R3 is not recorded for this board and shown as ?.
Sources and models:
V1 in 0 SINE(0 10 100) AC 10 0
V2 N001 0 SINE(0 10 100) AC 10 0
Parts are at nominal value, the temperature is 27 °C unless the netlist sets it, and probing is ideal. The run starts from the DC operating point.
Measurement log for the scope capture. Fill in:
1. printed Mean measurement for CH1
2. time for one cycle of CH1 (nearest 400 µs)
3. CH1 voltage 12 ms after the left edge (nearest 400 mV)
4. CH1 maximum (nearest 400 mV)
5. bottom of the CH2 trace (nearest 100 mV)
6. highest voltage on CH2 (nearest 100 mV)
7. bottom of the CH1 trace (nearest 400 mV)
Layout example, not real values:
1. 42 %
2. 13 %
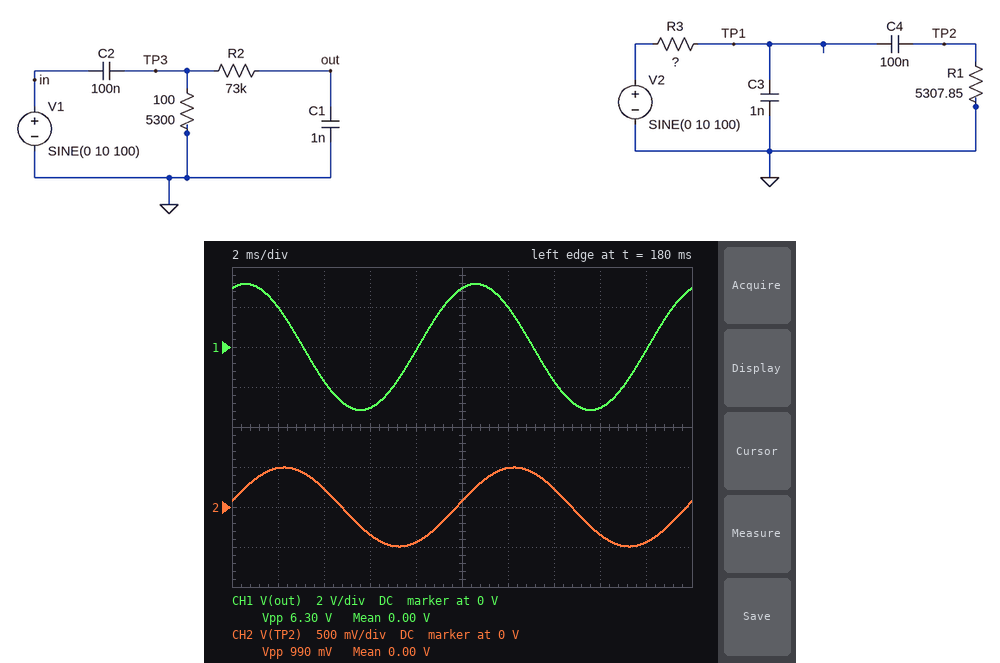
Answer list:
1. 0.00 V
2. 10.0 ms
3. 2.0 V
4. 3.2 V
5. -500 mV
6. 500 mV
7. -3.2 V
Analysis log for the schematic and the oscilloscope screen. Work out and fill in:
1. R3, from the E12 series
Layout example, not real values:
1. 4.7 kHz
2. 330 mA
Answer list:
1. 100 kΩ
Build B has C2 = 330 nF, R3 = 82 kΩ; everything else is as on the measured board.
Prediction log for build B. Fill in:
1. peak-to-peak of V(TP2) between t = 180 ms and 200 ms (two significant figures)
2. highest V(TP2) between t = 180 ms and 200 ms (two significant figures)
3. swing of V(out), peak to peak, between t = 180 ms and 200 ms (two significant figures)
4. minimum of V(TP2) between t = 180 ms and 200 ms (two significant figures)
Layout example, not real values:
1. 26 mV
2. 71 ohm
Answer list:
1. 1.2 V
2. 590 mV
3. 15 V
4. -590 mV
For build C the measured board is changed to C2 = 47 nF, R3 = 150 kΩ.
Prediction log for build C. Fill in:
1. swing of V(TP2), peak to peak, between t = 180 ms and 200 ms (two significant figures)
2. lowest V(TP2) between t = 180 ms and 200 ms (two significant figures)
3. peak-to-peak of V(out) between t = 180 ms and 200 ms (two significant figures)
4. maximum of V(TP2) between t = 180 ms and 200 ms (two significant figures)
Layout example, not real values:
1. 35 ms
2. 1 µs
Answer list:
1. 670 mV
2. -340 mV
3. 3.1 V
4. 340 mV
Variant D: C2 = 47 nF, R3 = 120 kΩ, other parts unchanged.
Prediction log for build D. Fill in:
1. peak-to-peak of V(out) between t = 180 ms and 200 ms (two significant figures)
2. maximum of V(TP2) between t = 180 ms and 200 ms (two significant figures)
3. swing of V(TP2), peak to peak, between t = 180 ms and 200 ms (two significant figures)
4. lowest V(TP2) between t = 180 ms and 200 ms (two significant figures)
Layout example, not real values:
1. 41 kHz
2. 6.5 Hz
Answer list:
1. 3.1 V
2. 420 mV
3. 830 mV
4. -420 mV
